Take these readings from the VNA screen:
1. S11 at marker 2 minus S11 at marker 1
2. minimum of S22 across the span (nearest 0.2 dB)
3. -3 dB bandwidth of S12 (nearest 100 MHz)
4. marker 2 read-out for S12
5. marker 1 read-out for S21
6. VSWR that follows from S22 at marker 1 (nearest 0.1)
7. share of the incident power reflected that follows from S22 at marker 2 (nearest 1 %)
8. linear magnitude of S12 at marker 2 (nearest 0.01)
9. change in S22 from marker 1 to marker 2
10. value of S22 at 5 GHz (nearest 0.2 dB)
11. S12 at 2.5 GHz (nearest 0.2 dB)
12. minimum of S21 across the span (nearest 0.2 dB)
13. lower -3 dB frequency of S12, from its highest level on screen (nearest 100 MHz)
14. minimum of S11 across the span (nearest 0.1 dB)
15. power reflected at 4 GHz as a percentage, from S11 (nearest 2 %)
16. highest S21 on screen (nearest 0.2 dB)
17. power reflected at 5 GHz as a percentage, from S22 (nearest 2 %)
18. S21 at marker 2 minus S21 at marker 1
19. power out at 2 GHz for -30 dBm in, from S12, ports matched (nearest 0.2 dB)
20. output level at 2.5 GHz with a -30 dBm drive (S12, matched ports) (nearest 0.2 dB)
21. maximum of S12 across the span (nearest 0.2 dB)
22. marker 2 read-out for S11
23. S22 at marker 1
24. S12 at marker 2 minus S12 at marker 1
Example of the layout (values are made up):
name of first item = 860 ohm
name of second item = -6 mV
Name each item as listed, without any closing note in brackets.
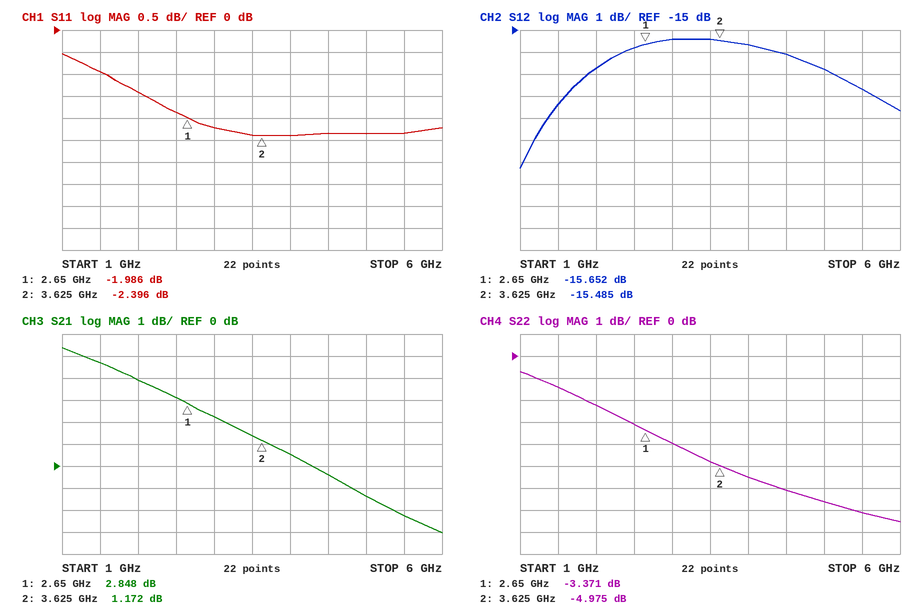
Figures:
S11 at marker 2 minus S11 at marker 1 = -0.410 dB
minimum of S22 across the span = -7.6 dB
-3 dB bandwidth of S12 = 4.4 GHz
marker 2 read-out for S12 = -15.485 dB
marker 1 read-out for S21 = 2.848 dB
VSWR that follows from S22 at marker 1 = 5.2
share of the incident power reflected that follows from S22 at marker 2 = 32 %
linear magnitude of S12 at marker 2 = 0.17
change in S22 from marker 1 to marker 2 = -1.604 dB
value of S22 at 5 GHz = -6.6 dB
S12 at 2.5 GHz = -15.8 dB
minimum of S21 across the span = -3.0 dB
lower -3 dB frequency of S12, from its highest level on screen = 1.5 GHz
minimum of S11 across the span = -2.4 dB
power reflected at 4 GHz as a percentage, from S11 = 58 %
highest S21 on screen = 5.4 dB
power reflected at 5 GHz as a percentage, from S22 = 22 %
S21 at marker 2 minus S21 at marker 1 = -1.676 dB
power out at 2 GHz for -30 dBm in, from S12, ports matched = -46.8 dBm
output level at 2.5 GHz with a -30 dBm drive (S12, matched ports) = -45.8 dBm
maximum of S12 across the span = -15.4 dB
marker 2 read-out for S11 = -2.396 dB
S22 at marker 1 = -3.371 dB
S12 at marker 2 minus S12 at marker 1 = 0.167 dB
